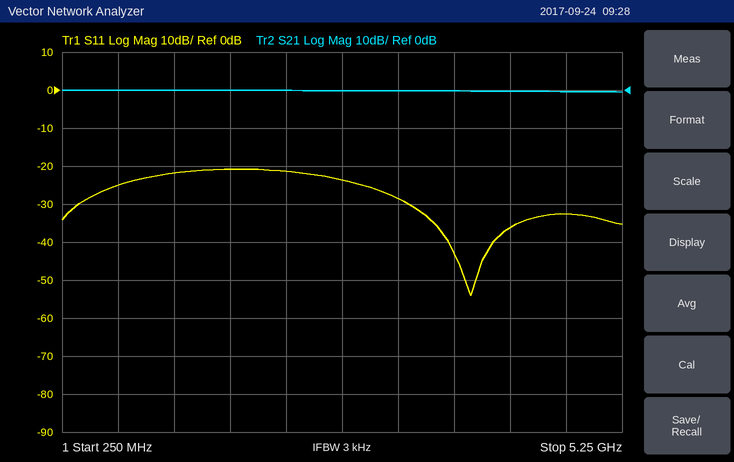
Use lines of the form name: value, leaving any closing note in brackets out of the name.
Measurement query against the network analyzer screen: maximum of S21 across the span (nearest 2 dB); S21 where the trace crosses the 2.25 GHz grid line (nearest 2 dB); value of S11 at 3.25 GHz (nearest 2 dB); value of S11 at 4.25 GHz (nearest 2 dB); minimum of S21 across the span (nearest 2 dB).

maximum of S21 across the span: 0 dB
S21 where the trace crosses the 2.25 GHz grid line: 0 dB
value of S11 at 3.25 GHz: -28 dB
value of S11 at 4.25 GHz: -36 dB
minimum of S21 across the span: 0 dB
